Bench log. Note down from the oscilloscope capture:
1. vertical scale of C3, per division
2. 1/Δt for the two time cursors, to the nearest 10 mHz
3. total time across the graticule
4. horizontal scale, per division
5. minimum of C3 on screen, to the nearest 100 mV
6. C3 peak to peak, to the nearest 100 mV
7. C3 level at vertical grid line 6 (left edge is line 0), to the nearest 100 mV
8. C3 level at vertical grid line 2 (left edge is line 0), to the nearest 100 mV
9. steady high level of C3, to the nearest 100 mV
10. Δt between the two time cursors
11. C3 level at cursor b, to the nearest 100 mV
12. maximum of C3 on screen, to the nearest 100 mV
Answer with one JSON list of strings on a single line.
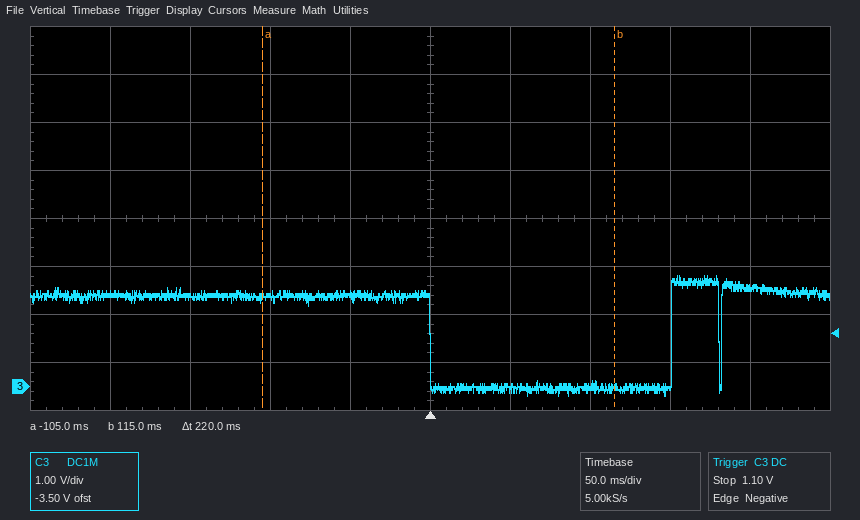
["1 V", "4.55 Hz", "500 ms", "50 ms", "-200 mV", "2.5 V", "0.0 V", "1.9 V", "1.9 V", "220 ms", "0.0 V", "2.3 V"]
